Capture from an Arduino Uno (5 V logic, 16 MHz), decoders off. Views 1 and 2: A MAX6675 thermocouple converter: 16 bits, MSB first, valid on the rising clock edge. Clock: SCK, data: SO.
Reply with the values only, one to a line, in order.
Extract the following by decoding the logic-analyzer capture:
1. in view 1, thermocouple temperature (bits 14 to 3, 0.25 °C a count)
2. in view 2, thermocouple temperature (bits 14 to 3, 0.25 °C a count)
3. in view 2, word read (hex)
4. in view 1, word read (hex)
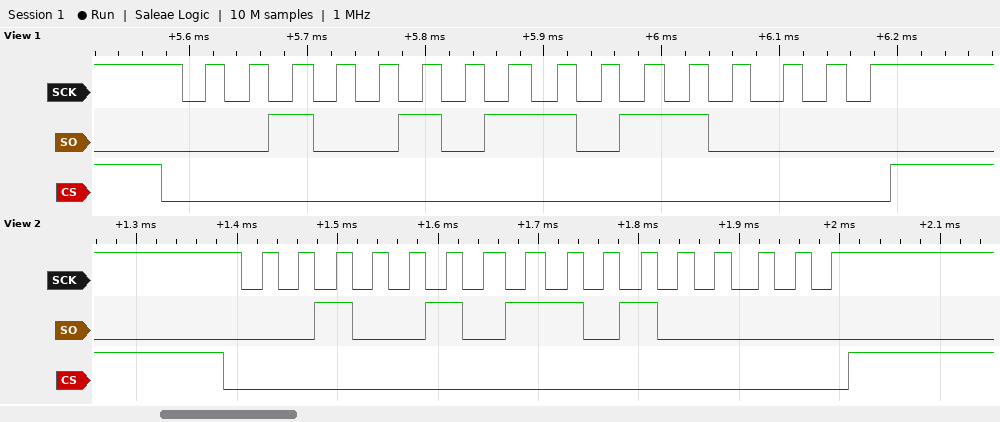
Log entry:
301.50 °C
301.00 °C
0x25A0
0x25B0
